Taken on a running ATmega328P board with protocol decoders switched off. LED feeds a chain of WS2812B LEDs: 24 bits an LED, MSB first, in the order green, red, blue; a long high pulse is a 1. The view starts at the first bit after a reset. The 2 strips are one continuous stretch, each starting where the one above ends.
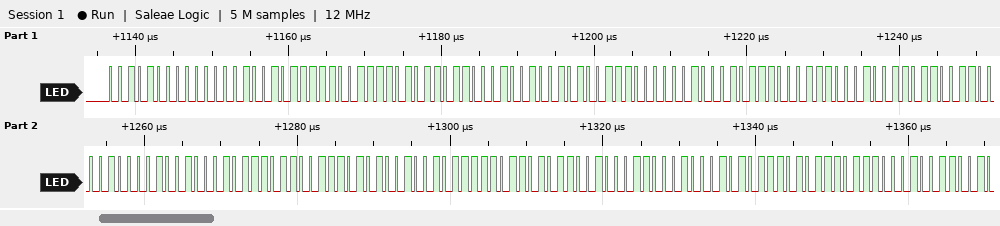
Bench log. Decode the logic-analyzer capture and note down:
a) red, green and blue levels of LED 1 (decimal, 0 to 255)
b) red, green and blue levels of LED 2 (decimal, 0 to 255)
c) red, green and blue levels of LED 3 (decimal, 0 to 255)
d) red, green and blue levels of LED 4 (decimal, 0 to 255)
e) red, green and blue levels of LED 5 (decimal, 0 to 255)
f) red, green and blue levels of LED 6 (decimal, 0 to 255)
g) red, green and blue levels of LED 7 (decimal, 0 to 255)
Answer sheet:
2, 40, 95
108, 61, 73
4, 78, 92
54, 113, 97
23, 9, 103
95, 82, 107
17, 35, 93
